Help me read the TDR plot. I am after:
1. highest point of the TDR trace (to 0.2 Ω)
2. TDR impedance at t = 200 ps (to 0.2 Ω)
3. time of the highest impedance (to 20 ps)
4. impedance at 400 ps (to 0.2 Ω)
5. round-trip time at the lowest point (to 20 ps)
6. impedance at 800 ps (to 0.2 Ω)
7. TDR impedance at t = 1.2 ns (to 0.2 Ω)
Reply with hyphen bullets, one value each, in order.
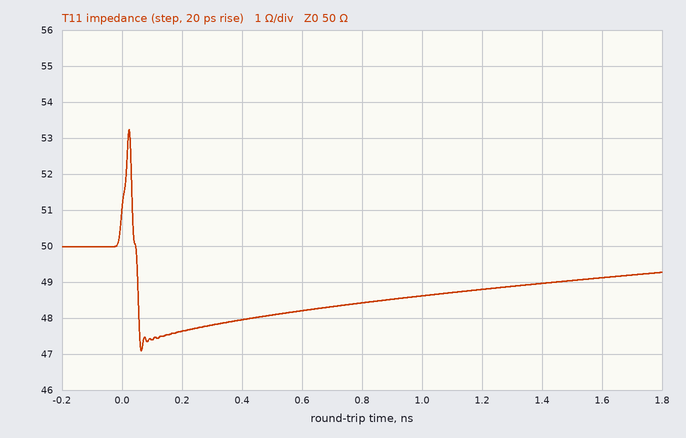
- 53.2 Ω
- 47.6 Ω
- 20 ps
- 48.0 Ω
- 60 ps
- 48.4 Ω
- 48.8 Ω
